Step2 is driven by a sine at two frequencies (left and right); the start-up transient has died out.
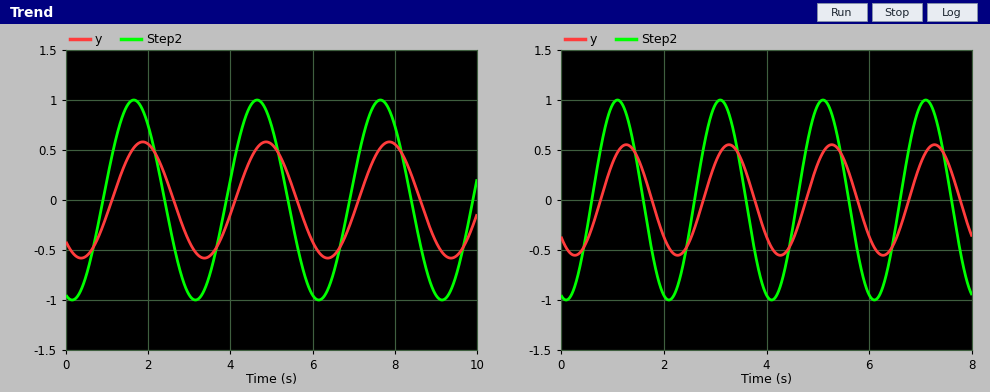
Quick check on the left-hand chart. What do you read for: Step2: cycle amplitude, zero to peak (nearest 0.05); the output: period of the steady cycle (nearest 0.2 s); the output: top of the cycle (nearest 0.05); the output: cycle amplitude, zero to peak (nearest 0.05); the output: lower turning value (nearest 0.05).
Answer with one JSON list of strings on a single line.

["1.00", "3.0 s", "0.60", "0.60", "-0.60"]
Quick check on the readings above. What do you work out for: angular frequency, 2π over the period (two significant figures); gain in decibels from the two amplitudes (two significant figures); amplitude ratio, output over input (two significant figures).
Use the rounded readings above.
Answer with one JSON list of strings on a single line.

["2.1 rad/s", "-4.4 dB", "0.60"]
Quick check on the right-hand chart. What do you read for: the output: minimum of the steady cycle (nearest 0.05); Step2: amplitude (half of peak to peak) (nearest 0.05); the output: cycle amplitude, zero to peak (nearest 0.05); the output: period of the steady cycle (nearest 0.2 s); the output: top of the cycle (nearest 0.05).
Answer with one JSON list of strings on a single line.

["-0.55", "1.00", "0.55", "2.0 s", "0.55"]
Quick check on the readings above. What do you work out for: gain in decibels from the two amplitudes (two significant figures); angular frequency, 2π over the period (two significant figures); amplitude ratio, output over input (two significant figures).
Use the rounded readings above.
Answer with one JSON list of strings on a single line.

["-5.2 dB", "3.1 rad/s", "0.55"]
